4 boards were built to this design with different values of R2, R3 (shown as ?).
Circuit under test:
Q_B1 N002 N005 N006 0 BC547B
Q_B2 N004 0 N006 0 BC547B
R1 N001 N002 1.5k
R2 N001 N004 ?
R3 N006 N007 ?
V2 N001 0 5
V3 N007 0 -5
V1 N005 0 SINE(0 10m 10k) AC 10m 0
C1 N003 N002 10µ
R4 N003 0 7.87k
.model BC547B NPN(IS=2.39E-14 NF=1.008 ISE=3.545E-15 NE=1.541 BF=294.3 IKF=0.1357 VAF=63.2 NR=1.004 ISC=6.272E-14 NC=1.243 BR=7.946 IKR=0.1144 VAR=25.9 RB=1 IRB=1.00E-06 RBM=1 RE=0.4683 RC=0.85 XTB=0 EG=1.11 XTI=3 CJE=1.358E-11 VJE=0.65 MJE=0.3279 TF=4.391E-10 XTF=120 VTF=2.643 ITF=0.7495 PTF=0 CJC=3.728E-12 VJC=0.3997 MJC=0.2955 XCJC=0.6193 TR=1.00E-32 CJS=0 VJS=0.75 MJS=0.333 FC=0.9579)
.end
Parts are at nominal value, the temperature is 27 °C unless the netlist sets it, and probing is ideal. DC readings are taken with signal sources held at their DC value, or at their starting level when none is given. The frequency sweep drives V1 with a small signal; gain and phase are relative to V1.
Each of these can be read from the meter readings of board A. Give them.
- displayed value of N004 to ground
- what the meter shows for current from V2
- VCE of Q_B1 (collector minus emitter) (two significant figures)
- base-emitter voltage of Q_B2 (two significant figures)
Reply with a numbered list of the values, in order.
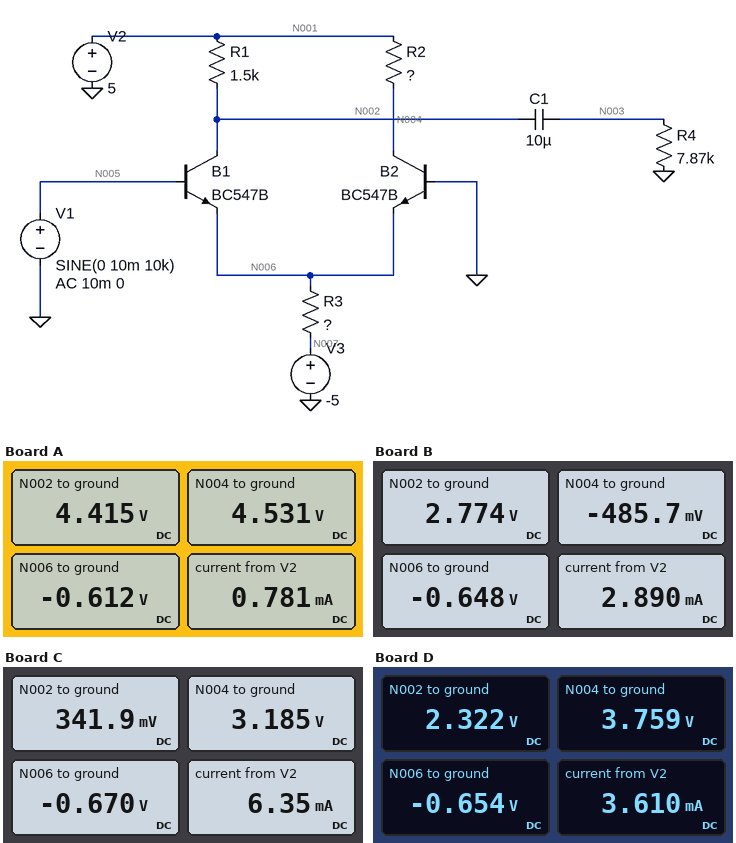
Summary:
1. 4.531 V
2. 0.781 mA
3. 5.0 V
4. 610 mV
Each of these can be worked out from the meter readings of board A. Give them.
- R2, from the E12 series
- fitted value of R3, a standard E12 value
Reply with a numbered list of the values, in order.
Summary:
1. 1.2 kΩ
2. 5.6 kΩ
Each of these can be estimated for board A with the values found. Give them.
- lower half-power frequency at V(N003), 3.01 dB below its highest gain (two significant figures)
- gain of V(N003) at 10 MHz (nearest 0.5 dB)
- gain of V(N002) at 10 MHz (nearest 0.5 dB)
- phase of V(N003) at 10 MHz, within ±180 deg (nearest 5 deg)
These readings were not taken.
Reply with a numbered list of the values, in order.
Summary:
1. 1.7 Hz
2. 19.5 dB
3. 19.5 dB
4. 170 deg
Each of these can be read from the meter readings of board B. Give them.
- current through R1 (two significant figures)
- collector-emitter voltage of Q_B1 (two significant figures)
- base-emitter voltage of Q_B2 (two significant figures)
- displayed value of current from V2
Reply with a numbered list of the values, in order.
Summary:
1. 1.5 mA
2. 3.4 V
3. 650 mV
4. 2.890 mA
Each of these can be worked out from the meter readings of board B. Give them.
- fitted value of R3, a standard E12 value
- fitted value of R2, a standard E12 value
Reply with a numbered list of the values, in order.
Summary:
1. 1.5 kΩ
2. 3.9 kΩ
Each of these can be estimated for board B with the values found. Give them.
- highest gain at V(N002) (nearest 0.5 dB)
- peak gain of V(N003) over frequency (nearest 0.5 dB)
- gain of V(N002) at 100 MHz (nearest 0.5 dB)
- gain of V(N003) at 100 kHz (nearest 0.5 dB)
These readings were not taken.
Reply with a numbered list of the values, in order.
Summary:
1. 30.0 dB
2. 30.0 dB
3. 25.0 dB
4. 28.5 dB
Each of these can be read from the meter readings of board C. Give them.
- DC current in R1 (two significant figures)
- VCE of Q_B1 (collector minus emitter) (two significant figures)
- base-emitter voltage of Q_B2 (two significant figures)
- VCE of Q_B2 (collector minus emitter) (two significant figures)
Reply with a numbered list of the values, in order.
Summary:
1. 3.1 mA
2. 1.0 V
3. 670 mV
4. 3.9 V
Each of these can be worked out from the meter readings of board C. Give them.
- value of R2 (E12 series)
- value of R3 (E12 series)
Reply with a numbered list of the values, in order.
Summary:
1. 560 Ω
2. 680 Ω
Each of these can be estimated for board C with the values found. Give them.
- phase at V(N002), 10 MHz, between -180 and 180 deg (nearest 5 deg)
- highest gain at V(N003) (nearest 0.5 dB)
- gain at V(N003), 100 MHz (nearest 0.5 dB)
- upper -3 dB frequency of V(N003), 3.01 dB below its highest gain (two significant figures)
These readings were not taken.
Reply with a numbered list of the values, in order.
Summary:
1. 165 deg
2. 36.5 dB
3. 28.0 dB
4. 40 MHz
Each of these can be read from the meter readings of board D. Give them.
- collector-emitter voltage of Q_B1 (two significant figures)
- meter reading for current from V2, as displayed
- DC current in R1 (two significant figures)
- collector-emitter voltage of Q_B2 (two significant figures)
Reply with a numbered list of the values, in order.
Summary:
1. 3.0 V
2. 3.610 mA
3. 1.8 mA
4. 4.4 V
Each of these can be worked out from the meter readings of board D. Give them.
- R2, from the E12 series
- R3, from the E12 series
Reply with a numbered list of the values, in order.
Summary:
1. 680 Ω
2. 1.2 kΩ
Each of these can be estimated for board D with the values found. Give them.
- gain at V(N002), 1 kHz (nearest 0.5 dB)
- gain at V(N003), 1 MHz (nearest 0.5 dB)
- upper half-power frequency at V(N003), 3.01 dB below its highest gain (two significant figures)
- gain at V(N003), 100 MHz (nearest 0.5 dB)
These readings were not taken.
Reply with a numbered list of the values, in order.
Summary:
1. 32.0 dB
2. 32.0 dB
3. 59 MHz
4. 26.5 dB
